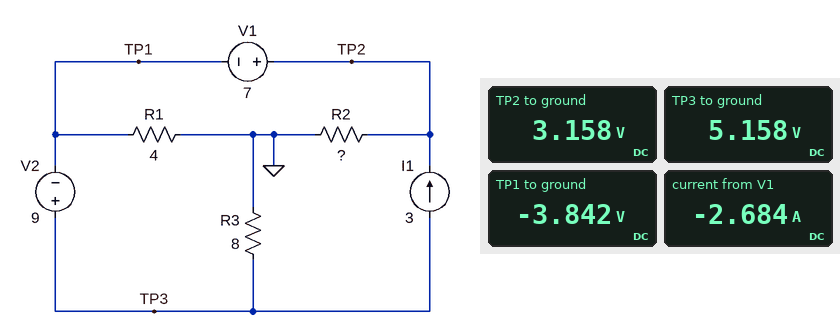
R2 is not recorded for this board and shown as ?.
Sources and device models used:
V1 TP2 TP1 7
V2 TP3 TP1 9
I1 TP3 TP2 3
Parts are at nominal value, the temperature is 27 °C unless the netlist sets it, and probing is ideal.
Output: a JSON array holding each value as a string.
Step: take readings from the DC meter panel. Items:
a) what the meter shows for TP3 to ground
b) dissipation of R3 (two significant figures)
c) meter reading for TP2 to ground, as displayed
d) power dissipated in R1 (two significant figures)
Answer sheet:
["5.158 V", "3.3 W", "3.158 V", "3.7 W"]
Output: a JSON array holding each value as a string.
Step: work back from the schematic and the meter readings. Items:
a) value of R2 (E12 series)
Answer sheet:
["10 Ω"]
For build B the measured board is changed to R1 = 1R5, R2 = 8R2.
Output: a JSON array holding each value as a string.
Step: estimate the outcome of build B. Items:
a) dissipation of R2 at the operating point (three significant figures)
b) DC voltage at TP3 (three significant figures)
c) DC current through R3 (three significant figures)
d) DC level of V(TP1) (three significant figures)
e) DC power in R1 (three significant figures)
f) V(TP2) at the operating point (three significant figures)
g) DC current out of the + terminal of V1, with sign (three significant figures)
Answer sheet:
["2.85 W", "6.83 V", "854 mA", "-2.17 V", "3.13 W", "4.83 V", "-2.41 A"]
